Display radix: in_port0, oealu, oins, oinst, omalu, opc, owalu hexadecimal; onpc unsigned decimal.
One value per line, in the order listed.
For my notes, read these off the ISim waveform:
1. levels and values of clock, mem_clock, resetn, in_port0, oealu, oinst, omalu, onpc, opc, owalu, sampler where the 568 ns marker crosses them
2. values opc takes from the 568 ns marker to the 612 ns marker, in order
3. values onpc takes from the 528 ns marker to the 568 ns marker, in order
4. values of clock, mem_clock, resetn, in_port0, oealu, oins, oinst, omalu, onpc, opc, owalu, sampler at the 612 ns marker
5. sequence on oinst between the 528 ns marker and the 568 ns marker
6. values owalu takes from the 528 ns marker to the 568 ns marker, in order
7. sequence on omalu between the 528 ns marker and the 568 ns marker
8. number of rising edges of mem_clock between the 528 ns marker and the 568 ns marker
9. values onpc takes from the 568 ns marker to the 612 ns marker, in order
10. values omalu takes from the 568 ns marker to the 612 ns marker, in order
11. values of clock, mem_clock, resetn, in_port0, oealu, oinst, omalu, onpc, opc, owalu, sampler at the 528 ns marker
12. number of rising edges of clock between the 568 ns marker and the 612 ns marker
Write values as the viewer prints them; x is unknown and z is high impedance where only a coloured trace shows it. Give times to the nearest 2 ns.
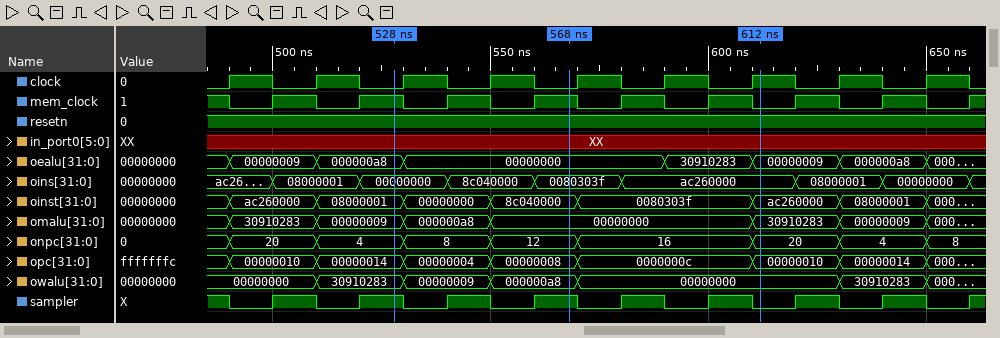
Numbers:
clock=0, mem_clock=1, resetn=1, in_port0=XX, oealu=00000000, oinst=8c040000, omalu=00000000, onpc=12, opc=00000008, owalu=000000a8, sampler=1
00000008, 0000000c, 00000010
4, 8, 12
clock=1, mem_clock=0, resetn=1, in_port0=XX, oealu=00000009, oins=ac260000, oinst=ac260000, omalu=30910283, onpc=20, opc=00000010, owalu=00000000, sampler=0
08000001, 00000000, 8c040000
30910283, 00000009, 000000a8
00000009, 000000a8, 00000000
2
12, 16, 20
00000000, 30910283
clock=0, mem_clock=1, resetn=1, in_port0=XX, oealu=000000a8, oinst=08000001, omalu=00000009, onpc=4, opc=00000014, owalu=30910283, sampler=1
3
